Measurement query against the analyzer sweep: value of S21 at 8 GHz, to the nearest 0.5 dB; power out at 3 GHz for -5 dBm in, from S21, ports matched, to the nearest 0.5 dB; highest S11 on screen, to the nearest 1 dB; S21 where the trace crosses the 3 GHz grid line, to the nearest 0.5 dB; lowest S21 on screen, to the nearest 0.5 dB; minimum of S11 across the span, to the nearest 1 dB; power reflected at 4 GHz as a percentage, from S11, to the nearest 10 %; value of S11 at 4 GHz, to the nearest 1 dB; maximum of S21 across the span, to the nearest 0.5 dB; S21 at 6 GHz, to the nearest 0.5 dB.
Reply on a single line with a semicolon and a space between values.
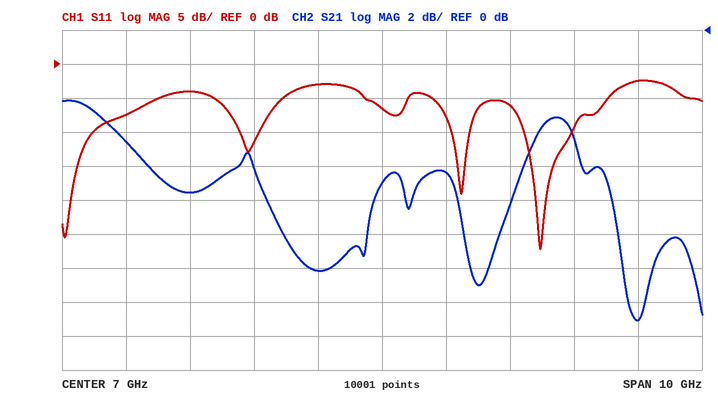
-8.5 dB; -11.5 dBm; -2 dB; -6.5 dB; -17.0 dB; -27 dB; 40 %; -4 dB; -4.0 dB; -14.0 dB
